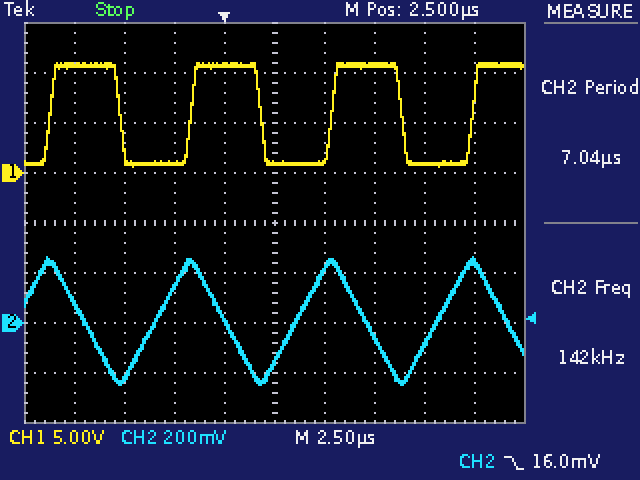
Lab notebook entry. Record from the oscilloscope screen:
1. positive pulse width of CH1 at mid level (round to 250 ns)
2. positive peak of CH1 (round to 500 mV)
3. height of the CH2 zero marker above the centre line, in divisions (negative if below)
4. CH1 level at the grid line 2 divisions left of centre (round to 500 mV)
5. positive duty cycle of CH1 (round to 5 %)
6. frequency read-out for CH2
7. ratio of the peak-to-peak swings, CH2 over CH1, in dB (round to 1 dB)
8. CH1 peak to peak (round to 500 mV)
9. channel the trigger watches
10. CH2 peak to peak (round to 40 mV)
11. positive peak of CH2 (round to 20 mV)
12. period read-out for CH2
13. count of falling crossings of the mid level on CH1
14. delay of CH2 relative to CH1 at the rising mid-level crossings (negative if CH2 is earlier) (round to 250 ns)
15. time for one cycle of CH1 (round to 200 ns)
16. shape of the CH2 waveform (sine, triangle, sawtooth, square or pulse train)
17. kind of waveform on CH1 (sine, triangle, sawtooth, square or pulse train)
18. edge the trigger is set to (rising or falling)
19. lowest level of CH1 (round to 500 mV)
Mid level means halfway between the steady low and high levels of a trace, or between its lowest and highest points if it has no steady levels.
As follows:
3.50 µs
11.0 V
-2.0 div
1.0 V
50 %
142 kHz
-26 dB
10.5 V
CH2
520 mV
260 mV
7.04 µs
3
-1.75 µs
7.0 µs
triangle
square
falling
500 mV
